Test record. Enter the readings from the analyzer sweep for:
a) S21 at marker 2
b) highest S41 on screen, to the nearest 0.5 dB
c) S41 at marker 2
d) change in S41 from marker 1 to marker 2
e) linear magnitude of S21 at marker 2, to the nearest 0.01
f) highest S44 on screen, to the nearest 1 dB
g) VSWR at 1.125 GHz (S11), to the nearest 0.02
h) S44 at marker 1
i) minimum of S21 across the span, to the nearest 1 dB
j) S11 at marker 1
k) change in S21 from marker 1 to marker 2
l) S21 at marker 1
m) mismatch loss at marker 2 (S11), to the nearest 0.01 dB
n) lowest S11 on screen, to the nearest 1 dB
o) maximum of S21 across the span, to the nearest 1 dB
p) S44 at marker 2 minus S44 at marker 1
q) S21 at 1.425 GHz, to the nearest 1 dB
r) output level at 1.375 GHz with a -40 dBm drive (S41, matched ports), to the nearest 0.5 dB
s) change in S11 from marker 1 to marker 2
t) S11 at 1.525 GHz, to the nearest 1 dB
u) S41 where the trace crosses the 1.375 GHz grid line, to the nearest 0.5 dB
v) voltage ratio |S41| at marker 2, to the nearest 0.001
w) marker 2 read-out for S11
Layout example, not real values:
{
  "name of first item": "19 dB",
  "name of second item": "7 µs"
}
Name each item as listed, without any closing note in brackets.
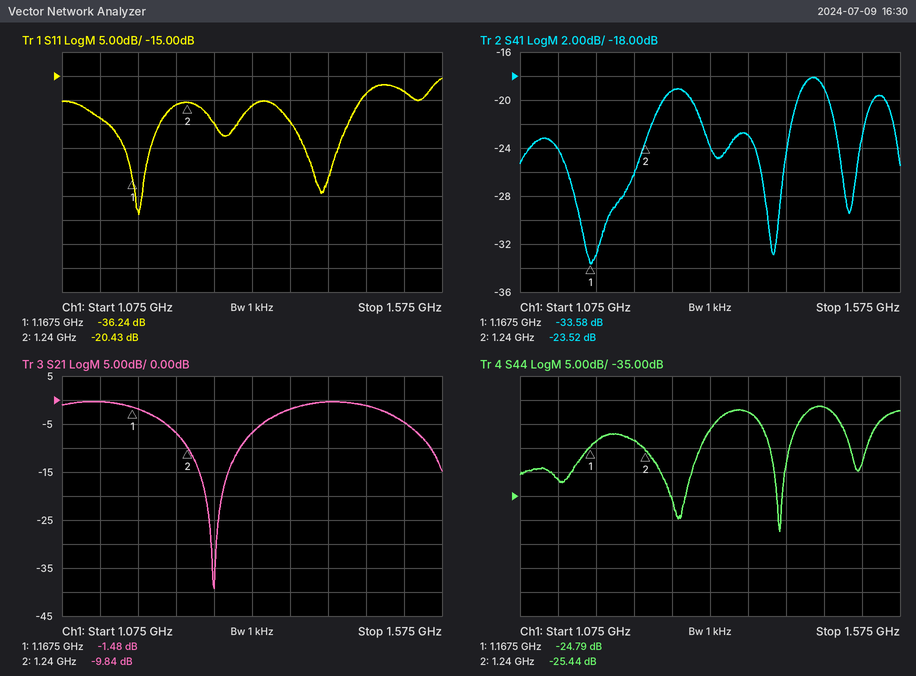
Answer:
{
  "S21 at marker 2": "-9.84 dB",
  "highest S41 on screen, to the nearest 0.5 dB": "-18.0 dB",
  "S41 at marker 2": "-23.52 dB",
  "change in S41 from marker 1 to marker 2": "10.06 dB",
  "linear magnitude of S21 at marker 2, to the nearest 0.01": "0.32",
  "highest S44 on screen, to the nearest 1 dB": "-16 dB",
  "VSWR at 1.125 GHz (S11), to the nearest 0.02": "1.14",
  "S44 at marker 1": "-24.79 dB",
  "minimum of S21 across the span, to the nearest 1 dB": "-39 dB",
  "S11 at marker 1": "-36.24 dB",
  "change in S21 from marker 1 to marker 2": "-8.36 dB",
  "S21 at marker 1": "-1.48 dB",
  "mismatch loss at marker 2 (S11), to the nearest 0.01 dB": "0.04 dB",
  "lowest S11 on screen, to the nearest 1 dB": "-44 dB",
  "maximum of S21 across the span, to the nearest 1 dB": "0 dB",
  "S44 at marker 2 minus S44 at marker 1": "-0.65 dB",
  "S21 at 1.425 GHz, to the nearest 1 dB": "0 dB",
  "output level at 1.375 GHz with a -40 dBm drive (S41, matched ports), to the nearest 0.5 dB": "-63.0 dBm",
  "change in S11 from marker 1 to marker 2": "15.81 dB",
  "S11 at 1.525 GHz, to the nearest 1 dB": "-18 dB",
  "S41 where the trace crosses the 1.375 GHz grid line, to the nearest 0.5 dB": "-23.0 dB",
  "voltage ratio |S41| at marker 2, to the nearest 0.001": "0.067",
  "marker 2 read-out for S11": "-20.43 dB"
}
